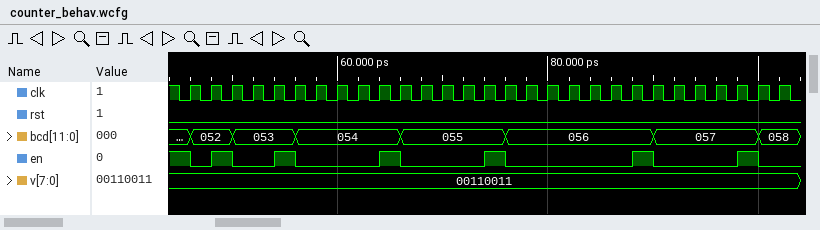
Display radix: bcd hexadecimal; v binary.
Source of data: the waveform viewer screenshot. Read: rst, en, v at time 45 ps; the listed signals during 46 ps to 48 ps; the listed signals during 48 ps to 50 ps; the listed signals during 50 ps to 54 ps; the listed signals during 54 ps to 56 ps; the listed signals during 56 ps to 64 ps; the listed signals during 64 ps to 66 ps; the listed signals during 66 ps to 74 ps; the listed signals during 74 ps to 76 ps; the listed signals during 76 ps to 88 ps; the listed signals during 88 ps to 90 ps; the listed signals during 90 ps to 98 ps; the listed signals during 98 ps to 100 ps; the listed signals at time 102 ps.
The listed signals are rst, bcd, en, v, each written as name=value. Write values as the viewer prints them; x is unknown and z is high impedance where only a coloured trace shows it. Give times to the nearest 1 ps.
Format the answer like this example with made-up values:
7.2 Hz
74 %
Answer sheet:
rst=0, en=1, v=00110011
rst=0, bcd=052, en=0, v=00110011
rst=0, bcd=052, en=1, v=00110011
rst=0, bcd=053, en=0, v=00110011
rst=0, bcd=053, en=1, v=00110011
rst=0, bcd=054, en=0, v=00110011
rst=0, bcd=054, en=1, v=00110011
rst=0, bcd=055, en=0, v=00110011
rst=0, bcd=055, en=1, v=00110011
rst=0, bcd=056, en=0, v=00110011
rst=0, bcd=056, en=1, v=00110011
rst=0, bcd=057, en=0, v=00110011
rst=0, bcd=057, en=1, v=00110011
rst=0, bcd=058, en=0, v=00110011
